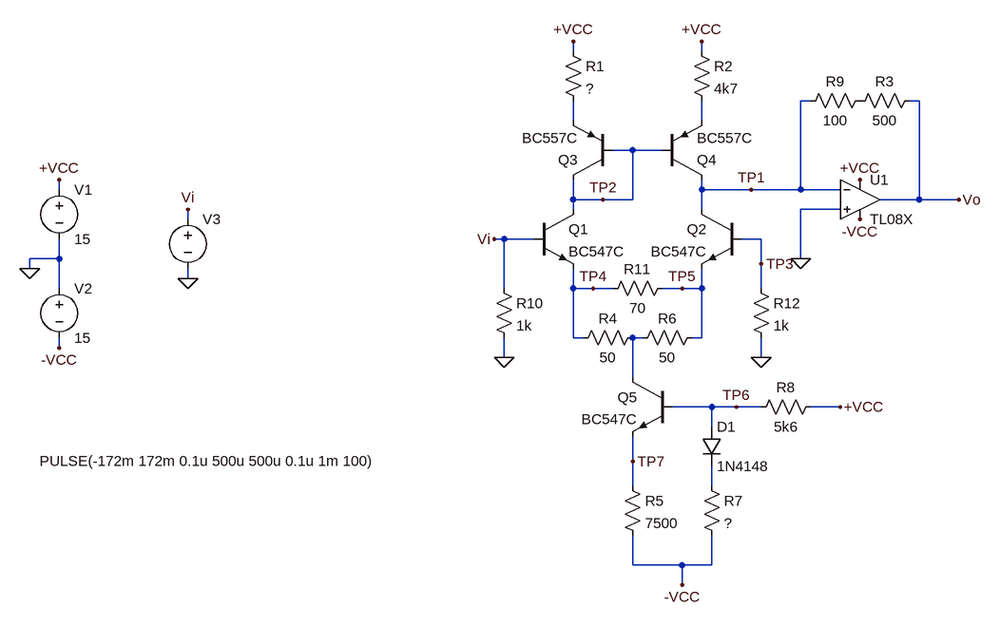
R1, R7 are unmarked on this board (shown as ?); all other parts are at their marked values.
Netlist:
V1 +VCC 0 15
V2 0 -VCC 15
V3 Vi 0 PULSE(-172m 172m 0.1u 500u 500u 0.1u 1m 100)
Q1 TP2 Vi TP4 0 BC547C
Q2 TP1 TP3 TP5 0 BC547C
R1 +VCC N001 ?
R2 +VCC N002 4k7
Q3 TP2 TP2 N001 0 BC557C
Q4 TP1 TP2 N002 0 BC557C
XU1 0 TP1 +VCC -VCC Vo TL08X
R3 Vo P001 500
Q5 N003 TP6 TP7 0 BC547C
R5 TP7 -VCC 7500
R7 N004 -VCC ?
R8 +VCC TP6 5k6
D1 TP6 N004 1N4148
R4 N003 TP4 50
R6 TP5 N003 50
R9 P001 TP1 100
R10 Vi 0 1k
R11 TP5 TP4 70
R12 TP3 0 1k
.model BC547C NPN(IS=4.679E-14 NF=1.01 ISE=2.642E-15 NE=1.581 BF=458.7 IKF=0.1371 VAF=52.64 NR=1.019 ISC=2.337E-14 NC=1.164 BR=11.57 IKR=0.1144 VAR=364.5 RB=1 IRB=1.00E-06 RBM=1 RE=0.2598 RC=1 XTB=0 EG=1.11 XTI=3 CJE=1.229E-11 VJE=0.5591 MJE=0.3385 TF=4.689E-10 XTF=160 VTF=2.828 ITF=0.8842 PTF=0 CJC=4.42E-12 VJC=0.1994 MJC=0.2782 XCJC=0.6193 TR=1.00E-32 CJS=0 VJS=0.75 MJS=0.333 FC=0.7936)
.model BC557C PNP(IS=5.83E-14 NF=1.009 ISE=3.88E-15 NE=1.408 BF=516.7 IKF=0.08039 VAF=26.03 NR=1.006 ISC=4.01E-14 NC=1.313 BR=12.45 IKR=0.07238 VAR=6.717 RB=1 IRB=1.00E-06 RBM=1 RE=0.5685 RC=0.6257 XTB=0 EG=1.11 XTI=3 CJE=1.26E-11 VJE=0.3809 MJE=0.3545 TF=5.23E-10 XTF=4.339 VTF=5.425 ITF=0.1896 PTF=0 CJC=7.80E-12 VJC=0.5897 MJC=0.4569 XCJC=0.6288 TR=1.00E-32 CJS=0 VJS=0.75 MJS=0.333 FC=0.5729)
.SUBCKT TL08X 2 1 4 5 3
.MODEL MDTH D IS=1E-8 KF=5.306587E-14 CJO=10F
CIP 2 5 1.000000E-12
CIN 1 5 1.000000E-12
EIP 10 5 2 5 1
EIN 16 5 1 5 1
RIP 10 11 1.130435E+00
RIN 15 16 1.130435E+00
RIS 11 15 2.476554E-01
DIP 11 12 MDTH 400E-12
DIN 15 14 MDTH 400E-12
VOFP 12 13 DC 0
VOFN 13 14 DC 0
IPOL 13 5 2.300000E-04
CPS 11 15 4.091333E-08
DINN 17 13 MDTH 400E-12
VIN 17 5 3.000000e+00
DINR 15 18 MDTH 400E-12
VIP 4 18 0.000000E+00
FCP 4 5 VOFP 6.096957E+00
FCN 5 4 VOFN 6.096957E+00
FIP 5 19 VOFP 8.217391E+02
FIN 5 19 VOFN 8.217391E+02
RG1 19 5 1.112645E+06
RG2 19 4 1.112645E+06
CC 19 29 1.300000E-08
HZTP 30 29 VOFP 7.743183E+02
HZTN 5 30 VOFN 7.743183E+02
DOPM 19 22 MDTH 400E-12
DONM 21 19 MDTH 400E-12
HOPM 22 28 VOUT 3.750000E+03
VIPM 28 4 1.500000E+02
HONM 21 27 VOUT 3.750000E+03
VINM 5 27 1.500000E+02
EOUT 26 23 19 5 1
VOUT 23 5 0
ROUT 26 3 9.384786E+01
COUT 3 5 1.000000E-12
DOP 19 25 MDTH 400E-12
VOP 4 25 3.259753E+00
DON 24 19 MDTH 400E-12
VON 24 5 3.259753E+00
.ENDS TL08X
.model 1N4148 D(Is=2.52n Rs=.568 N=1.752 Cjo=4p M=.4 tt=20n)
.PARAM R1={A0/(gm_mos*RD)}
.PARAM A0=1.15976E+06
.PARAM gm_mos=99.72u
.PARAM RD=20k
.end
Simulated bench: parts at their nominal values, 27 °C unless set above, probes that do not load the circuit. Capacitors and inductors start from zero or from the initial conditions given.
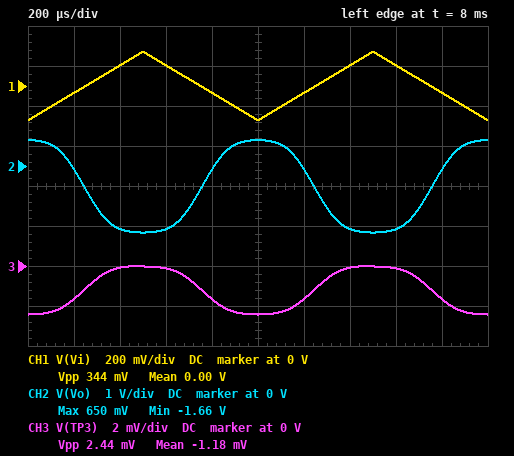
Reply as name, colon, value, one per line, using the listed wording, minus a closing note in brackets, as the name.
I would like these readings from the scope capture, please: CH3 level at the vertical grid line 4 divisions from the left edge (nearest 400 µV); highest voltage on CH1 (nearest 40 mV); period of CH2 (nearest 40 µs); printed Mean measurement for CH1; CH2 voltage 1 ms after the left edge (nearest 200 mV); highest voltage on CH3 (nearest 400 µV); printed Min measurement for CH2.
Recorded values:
CH3 level at the vertical grid line 4 divisions from the left edge: -1.6 mV
highest voltage on CH1: 160 mV
period of CH2: 1.00 ms
printed Mean measurement for CH1: 0.00 V
CH2 voltage 1 ms after the left edge: 600 mV
highest voltage on CH3: 0 V
printed Min measurement for CH2: -1.66 V
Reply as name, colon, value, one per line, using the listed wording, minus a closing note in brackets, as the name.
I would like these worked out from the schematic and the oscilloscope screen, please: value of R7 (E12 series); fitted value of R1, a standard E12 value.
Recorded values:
value of R7: 2.2 kΩ
fitted value of R1, a standard E12 value: 12 kΩ
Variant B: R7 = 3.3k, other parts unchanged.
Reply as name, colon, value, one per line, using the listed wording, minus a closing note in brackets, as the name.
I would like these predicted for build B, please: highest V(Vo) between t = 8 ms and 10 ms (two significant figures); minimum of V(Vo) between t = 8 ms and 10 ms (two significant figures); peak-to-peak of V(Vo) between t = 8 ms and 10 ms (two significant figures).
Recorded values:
highest V(Vo) between t = 8 ms and 10 ms: 850 mV
minimum of V(Vo) between t = 8 ms and 10 ms: -1.9 V
peak-to-peak of V(Vo) between t = 8 ms and 10 ms: 2.7 V
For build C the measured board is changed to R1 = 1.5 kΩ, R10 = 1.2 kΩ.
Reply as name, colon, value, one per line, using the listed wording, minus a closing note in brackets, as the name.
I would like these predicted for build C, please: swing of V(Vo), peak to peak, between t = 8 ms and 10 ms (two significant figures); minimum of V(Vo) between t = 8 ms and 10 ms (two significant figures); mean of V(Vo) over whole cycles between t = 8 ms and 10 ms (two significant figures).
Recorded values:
swing of V(Vo), peak to peak, between t = 8 ms and 10 ms: 870 mV
minimum of V(Vo) between t = 8 ms and 10 ms: -210 mV
mean of V(Vo) over whole cycles between t = 8 ms and 10 ms: 200 mV
